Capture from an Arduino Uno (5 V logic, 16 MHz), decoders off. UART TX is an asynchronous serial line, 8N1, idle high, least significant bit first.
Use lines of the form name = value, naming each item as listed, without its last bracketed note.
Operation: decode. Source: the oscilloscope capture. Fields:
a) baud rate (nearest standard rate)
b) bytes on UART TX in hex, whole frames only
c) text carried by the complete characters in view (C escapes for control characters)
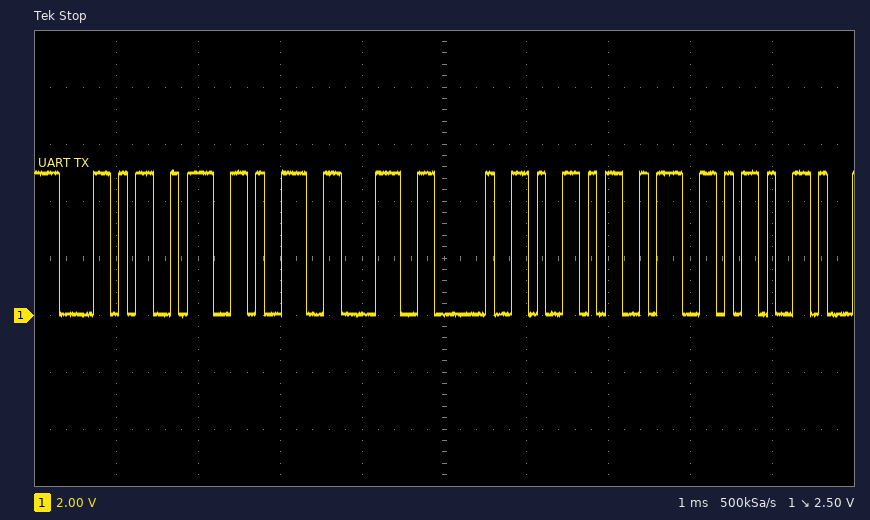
baud rate = 9600 baud
bytes on UART TX in hex, whole frames only = 0x58 0x3A 0x39 0x38 0x20 0x59 0x3A 0x2D
text carried by the complete characters in view = "X:98 Y:-"
